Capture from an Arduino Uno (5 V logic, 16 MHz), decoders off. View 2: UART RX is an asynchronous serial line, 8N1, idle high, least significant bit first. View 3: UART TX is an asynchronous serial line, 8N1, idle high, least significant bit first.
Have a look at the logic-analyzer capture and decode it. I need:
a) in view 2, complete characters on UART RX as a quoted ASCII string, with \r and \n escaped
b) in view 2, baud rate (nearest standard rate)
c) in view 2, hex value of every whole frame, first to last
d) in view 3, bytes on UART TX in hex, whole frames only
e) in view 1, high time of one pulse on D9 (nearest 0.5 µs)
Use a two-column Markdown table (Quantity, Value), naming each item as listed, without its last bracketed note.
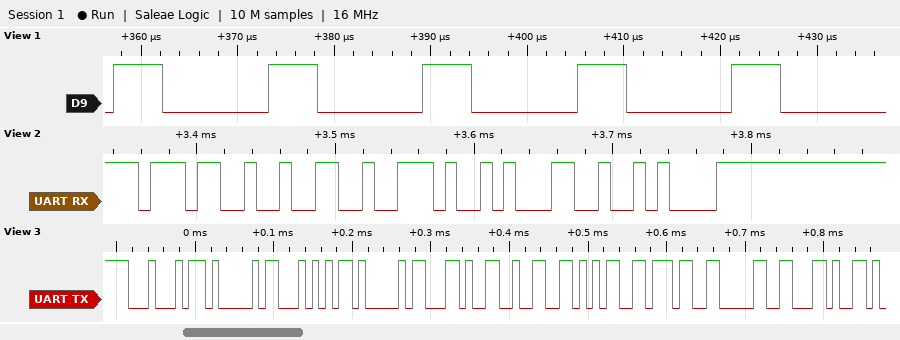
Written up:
| Quantity | Value |
|---|---|
| in view 2, complete characters on UART RX as a quoted ASCII string, with \r and \n escaped | "72.1\n" |
| in view 2, baud rate | 115200 baud |
| in view 2, hex value of every whole frame, first to last | 37 32 2E 31 0A |
| in view 3, bytes on UART TX in hex, whole frames only | 0x44 0x41 0x54 0x41 0x2C 0x32 0x35 0x37 0x30 0x2C |
| in view 1, high time of one pulse on D9 | 5.0 µs |
